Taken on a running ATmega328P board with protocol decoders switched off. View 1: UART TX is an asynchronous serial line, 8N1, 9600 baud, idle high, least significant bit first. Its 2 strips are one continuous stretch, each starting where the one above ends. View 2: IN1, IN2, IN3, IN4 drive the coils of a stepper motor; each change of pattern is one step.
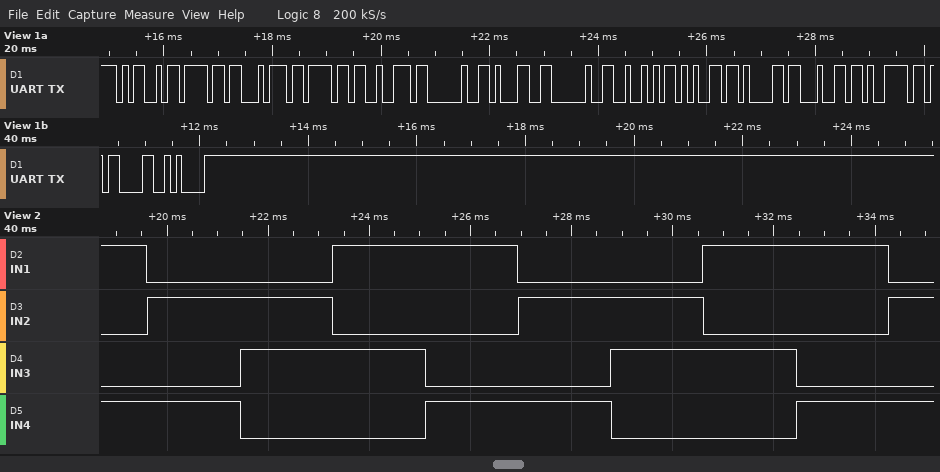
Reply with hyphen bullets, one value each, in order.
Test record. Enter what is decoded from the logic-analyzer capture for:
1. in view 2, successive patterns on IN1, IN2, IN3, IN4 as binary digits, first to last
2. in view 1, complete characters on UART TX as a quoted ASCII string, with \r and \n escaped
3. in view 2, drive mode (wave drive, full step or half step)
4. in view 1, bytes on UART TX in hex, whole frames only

- 1001 0101 0110 1010 1001 0101 0110 1010 1001 0101
- "Motor 1 Ready\r\n"
- full step
- 4D 6F 74 6F 72 20 31 20 52 65 61 64 79 0D 0A
